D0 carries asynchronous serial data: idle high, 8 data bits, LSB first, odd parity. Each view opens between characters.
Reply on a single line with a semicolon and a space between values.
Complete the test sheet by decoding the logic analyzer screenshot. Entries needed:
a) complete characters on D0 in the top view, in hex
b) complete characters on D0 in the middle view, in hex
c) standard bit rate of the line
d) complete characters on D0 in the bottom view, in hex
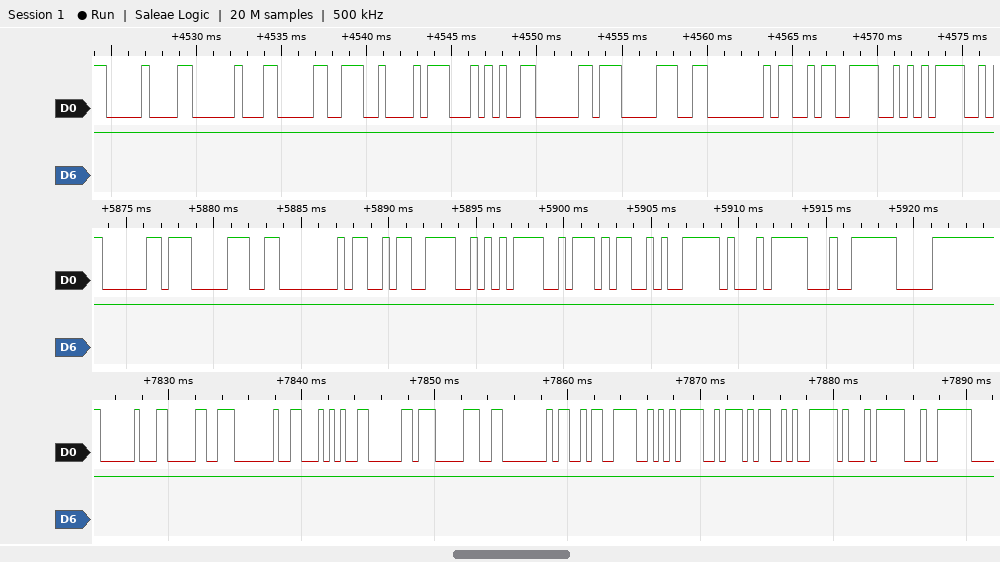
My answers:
10, 20, 30, 42, 54, 60, 70, 80, 9A, AA; 60, 70, 80, 9A, AA, BA, CA, D1, E4, F0; 2400 baud; 20, 30, 40, 54, 60, 70, 80, 9A, AA, BA, CA, D1, E4
